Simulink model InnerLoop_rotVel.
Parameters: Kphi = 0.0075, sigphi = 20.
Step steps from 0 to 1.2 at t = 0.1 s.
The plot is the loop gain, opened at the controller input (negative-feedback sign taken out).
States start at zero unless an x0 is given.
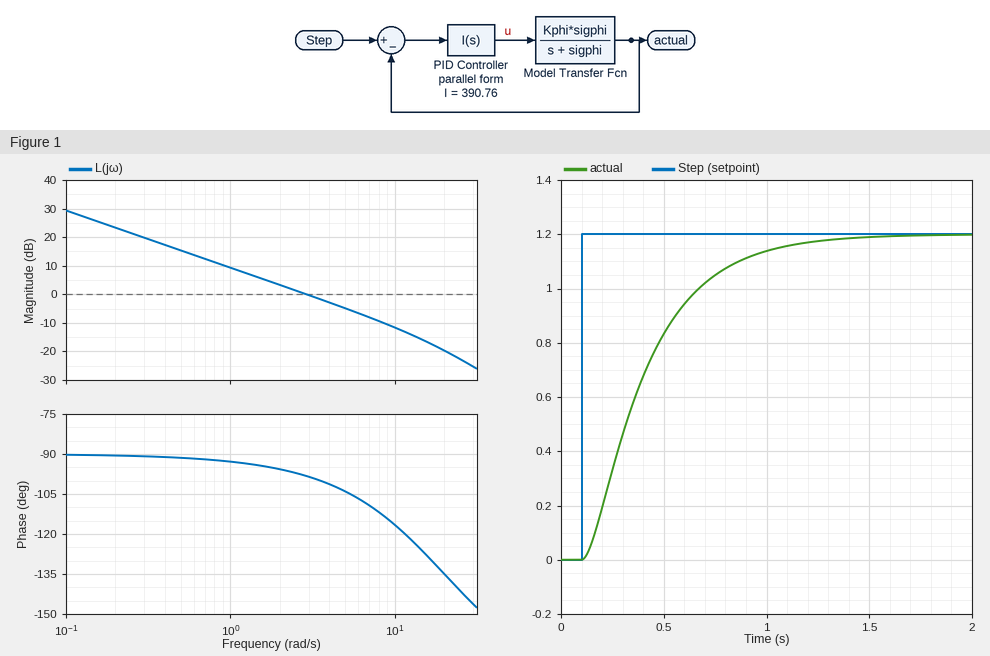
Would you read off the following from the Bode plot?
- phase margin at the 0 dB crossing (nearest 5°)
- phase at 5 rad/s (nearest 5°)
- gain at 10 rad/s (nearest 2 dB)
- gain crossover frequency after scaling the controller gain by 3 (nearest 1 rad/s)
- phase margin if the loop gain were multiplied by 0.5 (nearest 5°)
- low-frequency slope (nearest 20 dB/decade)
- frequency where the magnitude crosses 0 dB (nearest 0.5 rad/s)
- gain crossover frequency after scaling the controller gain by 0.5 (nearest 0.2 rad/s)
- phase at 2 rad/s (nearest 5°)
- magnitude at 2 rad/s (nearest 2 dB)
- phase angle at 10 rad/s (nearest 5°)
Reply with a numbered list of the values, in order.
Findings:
1. 80°
2. -105°
3. -12 dB
4. 8 rad/s
5. 85°
6. -20 dB/decade
7. 3.0 rad/s
8. 1.4 rad/s
9. -95°
10. 4 dB
11. -115°
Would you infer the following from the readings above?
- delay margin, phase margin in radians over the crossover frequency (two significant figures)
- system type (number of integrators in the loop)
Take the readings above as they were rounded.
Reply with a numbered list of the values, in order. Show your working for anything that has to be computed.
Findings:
1. 80 × π / 180 / 3 = 0.47 s
2. 1
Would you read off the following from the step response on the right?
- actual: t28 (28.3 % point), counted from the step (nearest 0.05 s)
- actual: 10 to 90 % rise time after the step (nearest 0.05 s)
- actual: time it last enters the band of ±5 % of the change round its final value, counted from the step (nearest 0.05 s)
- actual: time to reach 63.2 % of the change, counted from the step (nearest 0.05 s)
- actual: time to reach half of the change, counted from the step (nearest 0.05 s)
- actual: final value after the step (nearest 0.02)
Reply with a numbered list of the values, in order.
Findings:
1. 0.15 s
2. 0.65 s
3. 0.90 s
4. 0.35 s
5. 0.25 s
6. 1.20
